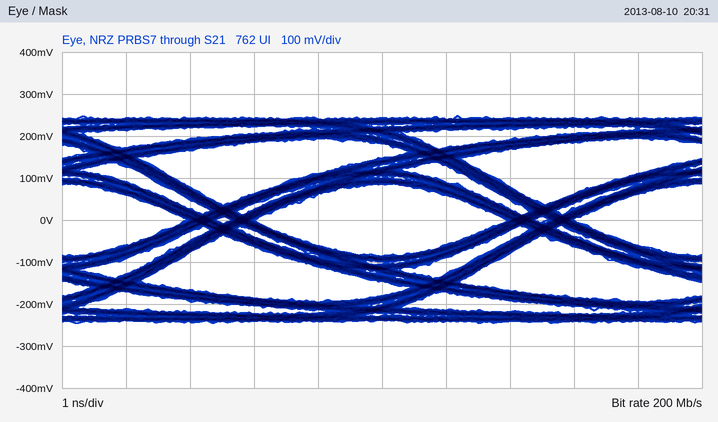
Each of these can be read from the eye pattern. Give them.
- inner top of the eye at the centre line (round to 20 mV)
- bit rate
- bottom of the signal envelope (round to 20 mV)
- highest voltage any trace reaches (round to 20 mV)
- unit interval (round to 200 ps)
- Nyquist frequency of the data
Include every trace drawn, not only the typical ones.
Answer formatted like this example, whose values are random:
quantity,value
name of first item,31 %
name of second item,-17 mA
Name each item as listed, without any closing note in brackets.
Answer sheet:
quantity,value
inner top of the eye at the centre line,80 mV
bit rate,200 Mb/s
bottom of the signal envelope,-240 mV
highest voltage any trace reaches,240 mV
unit interval,5.0 ns
Nyquist frequency of the data,100 MHz
